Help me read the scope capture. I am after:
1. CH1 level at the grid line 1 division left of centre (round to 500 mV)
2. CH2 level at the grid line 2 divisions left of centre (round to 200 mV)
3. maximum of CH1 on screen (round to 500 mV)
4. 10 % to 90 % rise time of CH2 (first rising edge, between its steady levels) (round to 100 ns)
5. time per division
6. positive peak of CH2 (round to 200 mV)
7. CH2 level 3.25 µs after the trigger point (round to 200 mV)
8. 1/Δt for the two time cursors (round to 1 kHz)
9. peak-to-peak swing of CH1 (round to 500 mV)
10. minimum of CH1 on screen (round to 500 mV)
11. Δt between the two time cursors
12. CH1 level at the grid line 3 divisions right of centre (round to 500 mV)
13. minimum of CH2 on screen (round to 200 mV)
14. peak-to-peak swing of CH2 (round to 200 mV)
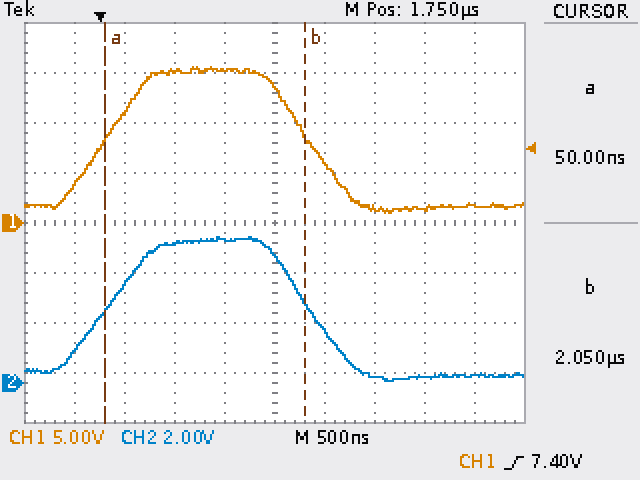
15.5 V
5.6 V
15.5 V
800 ns
500 ns
5.8 V
200 mV
500 kHz
14.5 V
1.0 V
2.00 µs
1.5 V
0.0 V
5.8 V
